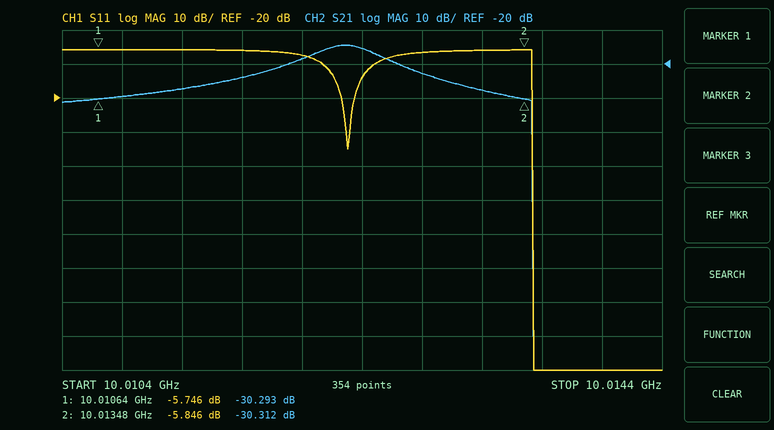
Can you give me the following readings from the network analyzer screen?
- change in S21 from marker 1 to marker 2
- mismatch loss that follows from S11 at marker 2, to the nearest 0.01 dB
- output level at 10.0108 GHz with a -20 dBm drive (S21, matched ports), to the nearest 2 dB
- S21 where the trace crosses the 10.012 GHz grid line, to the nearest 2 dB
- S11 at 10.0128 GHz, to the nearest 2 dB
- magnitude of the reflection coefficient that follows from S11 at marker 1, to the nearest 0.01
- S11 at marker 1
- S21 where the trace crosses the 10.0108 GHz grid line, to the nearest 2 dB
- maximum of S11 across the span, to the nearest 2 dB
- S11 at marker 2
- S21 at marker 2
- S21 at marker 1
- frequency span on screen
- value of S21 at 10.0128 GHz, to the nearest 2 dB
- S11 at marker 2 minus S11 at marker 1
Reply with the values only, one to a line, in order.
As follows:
-0.019 dB
1.31 dB
-50 dBm
-18 dB
-6 dB
0.52
-5.746 dB
-30 dB
-6 dB
-5.846 dB
-30.312 dB
-30.293 dB
4 MHz
-22 dB
-0.100 dB
